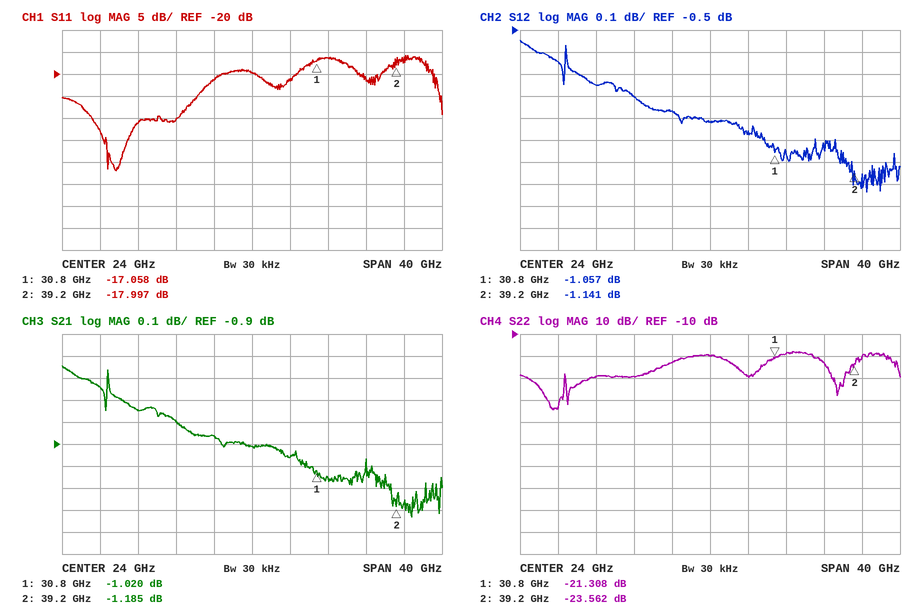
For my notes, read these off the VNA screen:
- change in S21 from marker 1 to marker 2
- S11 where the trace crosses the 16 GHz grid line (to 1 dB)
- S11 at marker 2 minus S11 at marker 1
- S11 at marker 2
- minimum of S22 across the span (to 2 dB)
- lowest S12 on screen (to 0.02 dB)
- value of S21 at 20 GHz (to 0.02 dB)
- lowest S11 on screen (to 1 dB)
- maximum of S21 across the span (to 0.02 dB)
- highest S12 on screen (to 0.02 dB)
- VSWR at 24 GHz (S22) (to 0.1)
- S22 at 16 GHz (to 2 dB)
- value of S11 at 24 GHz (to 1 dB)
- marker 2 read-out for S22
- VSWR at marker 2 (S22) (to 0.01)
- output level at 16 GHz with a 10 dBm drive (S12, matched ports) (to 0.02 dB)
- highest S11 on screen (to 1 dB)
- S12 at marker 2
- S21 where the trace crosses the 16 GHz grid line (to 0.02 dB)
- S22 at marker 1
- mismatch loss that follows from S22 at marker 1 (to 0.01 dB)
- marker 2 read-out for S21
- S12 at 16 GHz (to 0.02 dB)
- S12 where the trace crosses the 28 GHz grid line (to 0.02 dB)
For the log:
-0.165 dB
-30 dB
-0.939 dB
-17.997 dB
-44 dB
-1.24 dB
-0.86 dB
-42 dB
-0.54 dB
-0.54 dB
1.2
-30 dB
-20 dB
-23.562 dB
1.14
9.20 dBm
-16 dB
-1.141 dB
-0.80 dB
-21.308 dB
0.03 dB
-1.185 dB
-0.80 dB
-0.96 dB
